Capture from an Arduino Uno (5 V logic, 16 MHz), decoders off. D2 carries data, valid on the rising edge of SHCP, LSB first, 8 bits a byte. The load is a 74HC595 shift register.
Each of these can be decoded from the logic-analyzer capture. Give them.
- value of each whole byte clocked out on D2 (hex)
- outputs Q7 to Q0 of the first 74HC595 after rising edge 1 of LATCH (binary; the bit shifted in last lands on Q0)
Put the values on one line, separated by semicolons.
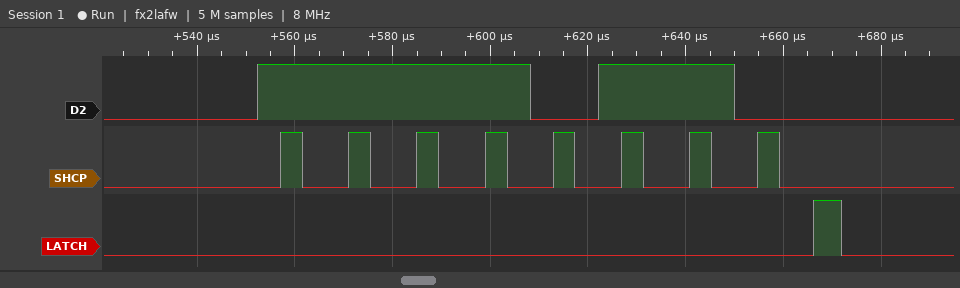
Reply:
6F; 11110110
